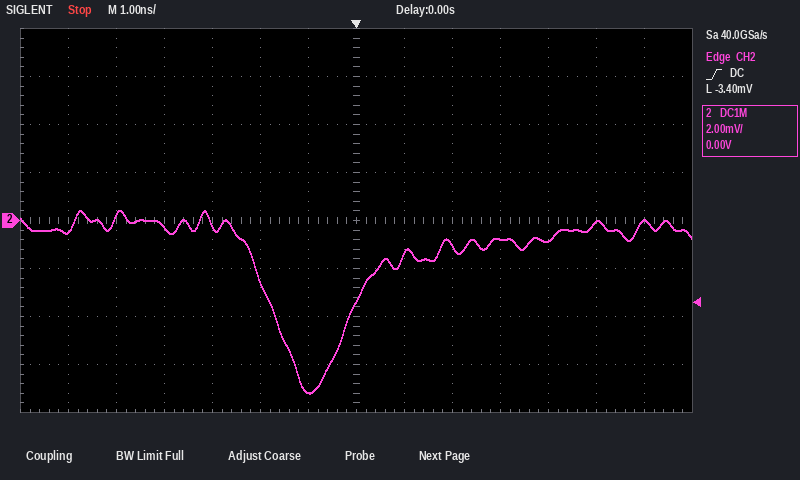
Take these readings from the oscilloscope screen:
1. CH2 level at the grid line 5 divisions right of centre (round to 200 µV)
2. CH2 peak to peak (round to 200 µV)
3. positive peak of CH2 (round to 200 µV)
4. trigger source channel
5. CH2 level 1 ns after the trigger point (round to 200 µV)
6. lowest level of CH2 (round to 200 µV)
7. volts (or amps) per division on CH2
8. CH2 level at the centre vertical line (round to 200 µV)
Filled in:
0.0 mV
7.6 mV
400 µV
CH2
-1.4 mV
-7.2 mV
2 mV
-3.4 mV
